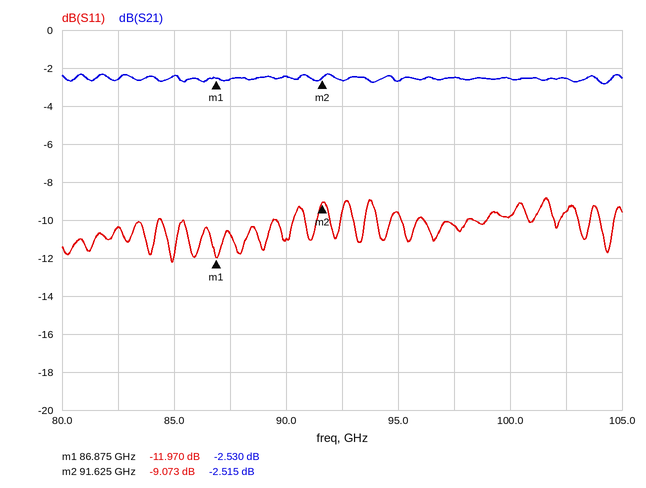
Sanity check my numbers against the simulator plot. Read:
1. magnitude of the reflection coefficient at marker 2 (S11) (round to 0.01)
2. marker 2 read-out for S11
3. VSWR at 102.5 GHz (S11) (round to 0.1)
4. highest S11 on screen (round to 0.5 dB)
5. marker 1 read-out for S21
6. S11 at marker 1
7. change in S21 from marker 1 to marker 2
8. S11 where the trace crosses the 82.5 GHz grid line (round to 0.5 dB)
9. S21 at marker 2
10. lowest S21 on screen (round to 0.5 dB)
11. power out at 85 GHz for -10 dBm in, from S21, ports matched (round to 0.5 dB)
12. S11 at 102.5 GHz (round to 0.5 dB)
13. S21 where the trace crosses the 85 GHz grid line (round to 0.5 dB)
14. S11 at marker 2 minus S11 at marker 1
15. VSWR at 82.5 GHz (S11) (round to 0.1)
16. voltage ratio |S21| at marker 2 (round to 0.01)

0.35
-9.073 dB
2.0
-9.0 dB
-2.530 dB
-11.970 dB
0.015 dB
-10.5 dB
-2.515 dB
-3.0 dB
-12.5 dBm
-9.5 dB
-2.5 dB
2.897 dB
1.9
0.75
